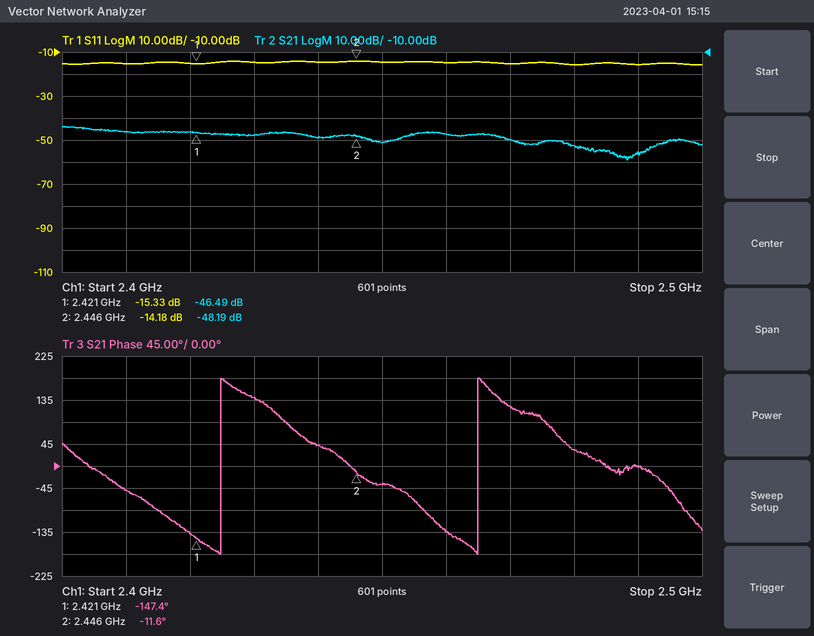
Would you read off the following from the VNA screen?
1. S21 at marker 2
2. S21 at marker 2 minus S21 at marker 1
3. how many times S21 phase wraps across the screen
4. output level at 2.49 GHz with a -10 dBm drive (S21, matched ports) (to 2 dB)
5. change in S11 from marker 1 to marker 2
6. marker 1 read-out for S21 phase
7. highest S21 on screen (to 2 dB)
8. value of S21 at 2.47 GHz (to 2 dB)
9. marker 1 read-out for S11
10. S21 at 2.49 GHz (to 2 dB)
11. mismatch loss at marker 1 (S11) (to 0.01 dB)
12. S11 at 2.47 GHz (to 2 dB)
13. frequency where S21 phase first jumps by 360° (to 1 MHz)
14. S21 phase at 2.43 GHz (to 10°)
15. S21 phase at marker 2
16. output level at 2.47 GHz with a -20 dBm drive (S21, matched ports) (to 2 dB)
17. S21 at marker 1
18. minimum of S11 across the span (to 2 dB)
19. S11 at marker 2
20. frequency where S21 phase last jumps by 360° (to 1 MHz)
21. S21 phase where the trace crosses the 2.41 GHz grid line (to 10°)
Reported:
-48.19 dB
-1.70 dB
2
-66 dBm
1.15 dB
-147.4°
-44 dB
-50 dB
-15.33 dB
-56 dB
0.13 dB
-16 dB
2.425 GHz
140°
-11.6°
-70 dBm
-46.49 dB
-16 dB
-14.18 dB
2.465 GHz
-50°
